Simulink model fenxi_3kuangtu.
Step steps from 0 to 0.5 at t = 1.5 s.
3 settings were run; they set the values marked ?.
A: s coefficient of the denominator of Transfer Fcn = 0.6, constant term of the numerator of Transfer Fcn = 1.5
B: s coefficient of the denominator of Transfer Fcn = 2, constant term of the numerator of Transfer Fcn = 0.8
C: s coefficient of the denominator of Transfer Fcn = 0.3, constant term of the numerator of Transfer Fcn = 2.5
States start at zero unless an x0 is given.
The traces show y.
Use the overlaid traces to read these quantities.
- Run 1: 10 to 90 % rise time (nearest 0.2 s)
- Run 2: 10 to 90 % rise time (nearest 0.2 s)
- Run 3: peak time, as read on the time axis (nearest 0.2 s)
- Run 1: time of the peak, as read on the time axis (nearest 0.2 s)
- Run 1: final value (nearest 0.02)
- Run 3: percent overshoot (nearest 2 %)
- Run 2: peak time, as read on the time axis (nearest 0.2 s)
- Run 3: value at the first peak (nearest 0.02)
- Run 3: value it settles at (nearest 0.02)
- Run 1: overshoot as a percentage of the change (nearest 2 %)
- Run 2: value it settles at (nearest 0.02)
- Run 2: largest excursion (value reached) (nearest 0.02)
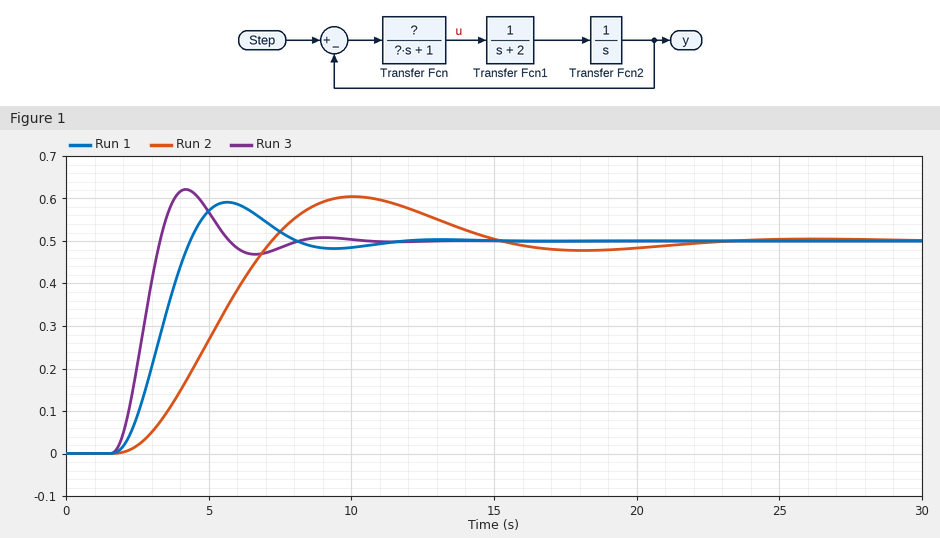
1.8 s
3.6 s
4.2 s
5.6 s
0.50
24 %
10.0 s
0.62
0.50
18 %
0.50
0.60
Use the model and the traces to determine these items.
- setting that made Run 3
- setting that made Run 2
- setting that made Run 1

C
B
A
